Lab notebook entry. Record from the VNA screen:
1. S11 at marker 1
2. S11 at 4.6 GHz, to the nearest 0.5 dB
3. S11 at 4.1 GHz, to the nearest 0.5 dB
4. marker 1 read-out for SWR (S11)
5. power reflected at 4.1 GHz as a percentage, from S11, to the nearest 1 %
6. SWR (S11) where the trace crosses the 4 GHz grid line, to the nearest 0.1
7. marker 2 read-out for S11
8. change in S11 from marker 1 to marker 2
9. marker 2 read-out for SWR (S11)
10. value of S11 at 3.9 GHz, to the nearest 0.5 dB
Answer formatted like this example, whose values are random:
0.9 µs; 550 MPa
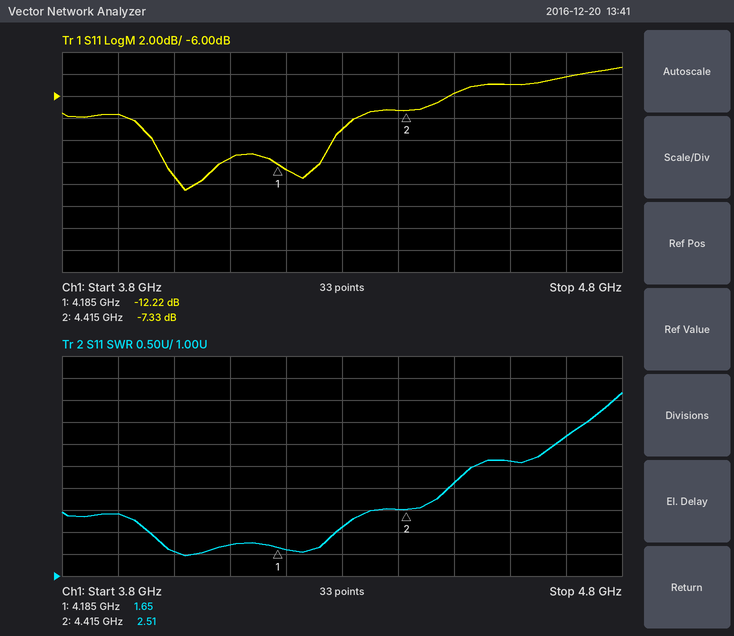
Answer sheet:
-12.22 dB; -5.0 dB; -11.5 dB; 1.65; 7 %; 1.6; -7.33 dB; 4.89 dB; 2.51; -7.5 dB
